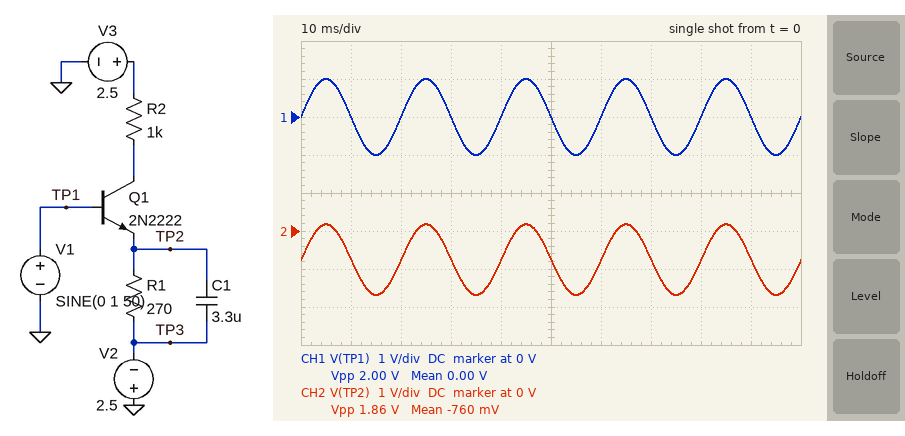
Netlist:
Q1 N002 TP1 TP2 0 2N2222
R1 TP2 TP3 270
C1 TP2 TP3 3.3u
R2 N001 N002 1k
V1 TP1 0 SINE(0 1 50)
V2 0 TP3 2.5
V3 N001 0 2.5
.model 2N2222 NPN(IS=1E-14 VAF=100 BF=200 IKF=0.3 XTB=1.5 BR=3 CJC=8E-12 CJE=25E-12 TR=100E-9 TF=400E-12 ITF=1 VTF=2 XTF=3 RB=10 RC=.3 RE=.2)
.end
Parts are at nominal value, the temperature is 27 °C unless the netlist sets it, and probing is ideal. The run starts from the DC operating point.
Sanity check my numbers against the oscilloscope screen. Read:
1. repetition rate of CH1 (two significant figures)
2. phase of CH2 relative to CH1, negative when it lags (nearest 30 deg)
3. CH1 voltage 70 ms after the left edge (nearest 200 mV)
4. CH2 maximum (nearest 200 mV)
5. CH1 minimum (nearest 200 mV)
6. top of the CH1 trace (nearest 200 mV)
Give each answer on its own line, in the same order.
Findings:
50 Hz
0 deg
0 V
200 mV
-1.0 V
1.0 V
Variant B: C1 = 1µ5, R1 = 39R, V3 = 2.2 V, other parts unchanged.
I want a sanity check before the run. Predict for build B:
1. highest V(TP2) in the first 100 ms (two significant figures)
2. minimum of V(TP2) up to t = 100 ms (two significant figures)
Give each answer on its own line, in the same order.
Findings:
-340 mV
-1.9 V
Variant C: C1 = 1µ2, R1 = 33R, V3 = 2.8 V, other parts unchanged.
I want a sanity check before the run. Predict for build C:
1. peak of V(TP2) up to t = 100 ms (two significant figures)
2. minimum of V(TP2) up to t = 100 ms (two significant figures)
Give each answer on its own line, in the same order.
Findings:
-410 mV
-1.9 V
